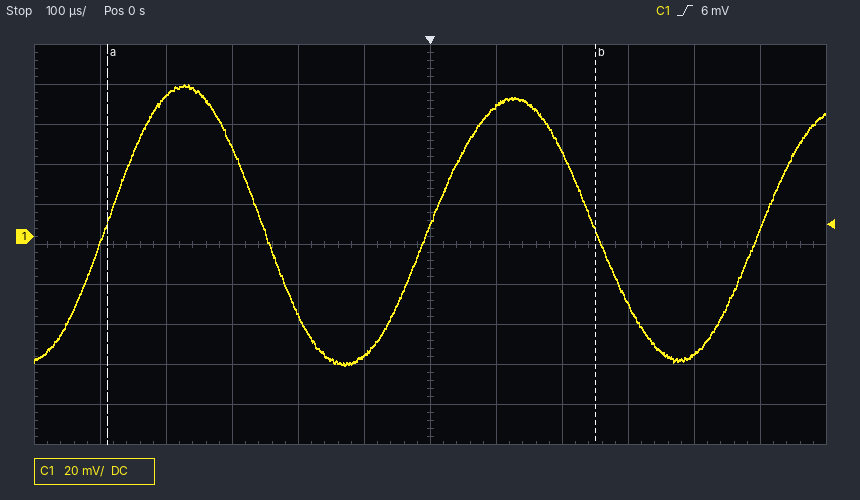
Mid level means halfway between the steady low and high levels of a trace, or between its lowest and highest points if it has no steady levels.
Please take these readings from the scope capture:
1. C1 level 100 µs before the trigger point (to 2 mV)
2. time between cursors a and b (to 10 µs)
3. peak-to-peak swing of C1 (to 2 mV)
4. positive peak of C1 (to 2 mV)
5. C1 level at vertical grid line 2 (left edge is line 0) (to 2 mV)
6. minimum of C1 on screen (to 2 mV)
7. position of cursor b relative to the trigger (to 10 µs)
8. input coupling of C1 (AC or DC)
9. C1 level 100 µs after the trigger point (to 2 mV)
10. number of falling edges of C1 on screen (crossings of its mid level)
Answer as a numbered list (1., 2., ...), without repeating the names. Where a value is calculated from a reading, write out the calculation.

1. -60 mV
2. 740 µs
3. 76 mV − (-64 mV) = 140 mV
4. 76 mV
5. 70 mV
6. -64 mV
7. +250 µs
8. DC
9. 66 mV
10. 2
